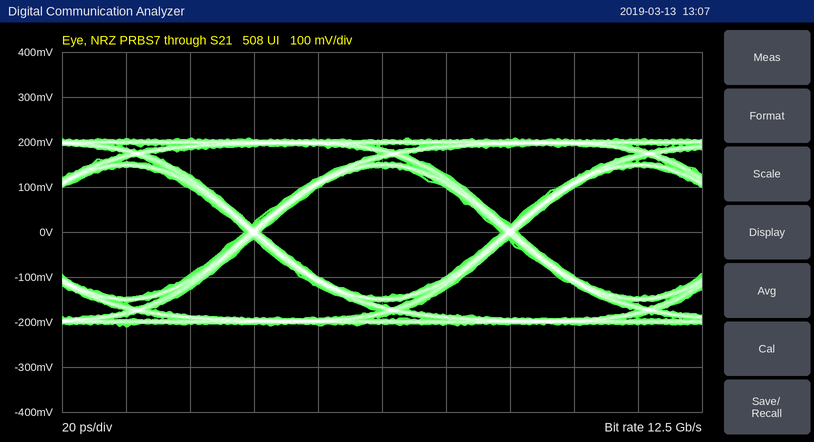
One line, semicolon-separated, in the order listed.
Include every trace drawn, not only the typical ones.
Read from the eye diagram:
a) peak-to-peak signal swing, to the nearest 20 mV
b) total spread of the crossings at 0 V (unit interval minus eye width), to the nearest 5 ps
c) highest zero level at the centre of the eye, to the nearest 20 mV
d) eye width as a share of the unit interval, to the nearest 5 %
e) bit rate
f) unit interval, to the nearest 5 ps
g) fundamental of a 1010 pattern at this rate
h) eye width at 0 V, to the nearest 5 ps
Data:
420 mV; 5 ps; -140 mV; 95 %; 12.5 Gb/s; 80 ps; 6.25 GHz; 75 ps
